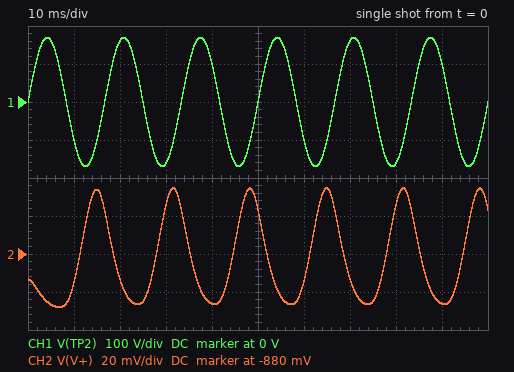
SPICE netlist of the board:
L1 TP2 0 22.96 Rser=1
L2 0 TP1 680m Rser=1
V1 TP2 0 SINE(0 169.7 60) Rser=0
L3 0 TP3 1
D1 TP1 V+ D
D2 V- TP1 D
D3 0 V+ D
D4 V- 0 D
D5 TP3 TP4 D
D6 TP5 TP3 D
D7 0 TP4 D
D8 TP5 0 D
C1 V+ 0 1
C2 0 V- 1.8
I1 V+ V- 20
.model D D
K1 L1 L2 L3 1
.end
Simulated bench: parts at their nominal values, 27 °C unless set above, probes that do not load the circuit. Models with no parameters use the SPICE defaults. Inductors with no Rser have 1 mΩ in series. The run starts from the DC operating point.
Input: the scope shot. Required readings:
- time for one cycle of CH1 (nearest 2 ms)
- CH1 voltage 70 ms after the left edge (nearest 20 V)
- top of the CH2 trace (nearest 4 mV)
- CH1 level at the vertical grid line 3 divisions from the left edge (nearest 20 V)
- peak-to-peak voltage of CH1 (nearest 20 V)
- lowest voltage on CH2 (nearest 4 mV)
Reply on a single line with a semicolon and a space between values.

16 ms; 160 V; -844 mV; -160 V; 340 V; -908 mV
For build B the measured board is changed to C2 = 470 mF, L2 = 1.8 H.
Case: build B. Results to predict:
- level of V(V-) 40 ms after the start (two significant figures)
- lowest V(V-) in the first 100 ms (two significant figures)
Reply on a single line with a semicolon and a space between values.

680 mV; 670 mV
